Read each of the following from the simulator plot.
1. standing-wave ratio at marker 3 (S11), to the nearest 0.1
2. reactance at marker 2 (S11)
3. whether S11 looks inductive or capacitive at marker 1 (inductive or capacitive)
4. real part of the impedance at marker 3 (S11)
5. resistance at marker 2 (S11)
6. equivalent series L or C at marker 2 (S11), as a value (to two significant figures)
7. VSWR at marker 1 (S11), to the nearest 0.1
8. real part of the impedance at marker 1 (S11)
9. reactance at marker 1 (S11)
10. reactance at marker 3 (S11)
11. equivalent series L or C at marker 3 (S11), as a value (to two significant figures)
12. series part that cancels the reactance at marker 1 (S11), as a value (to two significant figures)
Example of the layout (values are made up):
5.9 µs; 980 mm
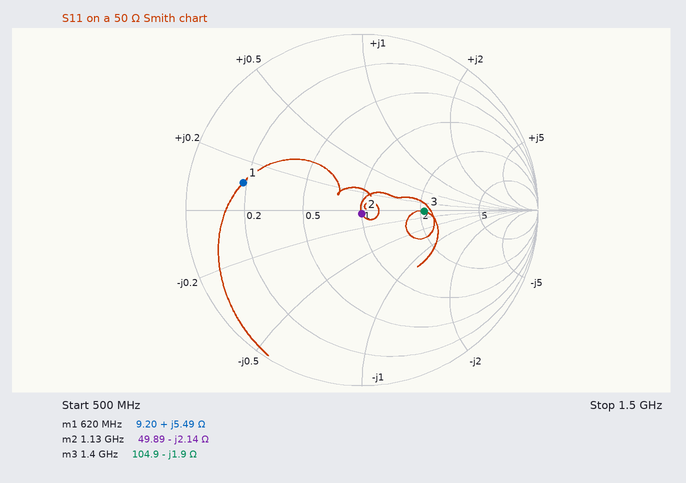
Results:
2.1; -2.14 Ω; inductive; 104.9 Ω; 49.89 Ω; 66 pF; 5.5; 9.20 Ω; +5.49 Ω; -1.9 Ω; 60 pF; 47 pF
